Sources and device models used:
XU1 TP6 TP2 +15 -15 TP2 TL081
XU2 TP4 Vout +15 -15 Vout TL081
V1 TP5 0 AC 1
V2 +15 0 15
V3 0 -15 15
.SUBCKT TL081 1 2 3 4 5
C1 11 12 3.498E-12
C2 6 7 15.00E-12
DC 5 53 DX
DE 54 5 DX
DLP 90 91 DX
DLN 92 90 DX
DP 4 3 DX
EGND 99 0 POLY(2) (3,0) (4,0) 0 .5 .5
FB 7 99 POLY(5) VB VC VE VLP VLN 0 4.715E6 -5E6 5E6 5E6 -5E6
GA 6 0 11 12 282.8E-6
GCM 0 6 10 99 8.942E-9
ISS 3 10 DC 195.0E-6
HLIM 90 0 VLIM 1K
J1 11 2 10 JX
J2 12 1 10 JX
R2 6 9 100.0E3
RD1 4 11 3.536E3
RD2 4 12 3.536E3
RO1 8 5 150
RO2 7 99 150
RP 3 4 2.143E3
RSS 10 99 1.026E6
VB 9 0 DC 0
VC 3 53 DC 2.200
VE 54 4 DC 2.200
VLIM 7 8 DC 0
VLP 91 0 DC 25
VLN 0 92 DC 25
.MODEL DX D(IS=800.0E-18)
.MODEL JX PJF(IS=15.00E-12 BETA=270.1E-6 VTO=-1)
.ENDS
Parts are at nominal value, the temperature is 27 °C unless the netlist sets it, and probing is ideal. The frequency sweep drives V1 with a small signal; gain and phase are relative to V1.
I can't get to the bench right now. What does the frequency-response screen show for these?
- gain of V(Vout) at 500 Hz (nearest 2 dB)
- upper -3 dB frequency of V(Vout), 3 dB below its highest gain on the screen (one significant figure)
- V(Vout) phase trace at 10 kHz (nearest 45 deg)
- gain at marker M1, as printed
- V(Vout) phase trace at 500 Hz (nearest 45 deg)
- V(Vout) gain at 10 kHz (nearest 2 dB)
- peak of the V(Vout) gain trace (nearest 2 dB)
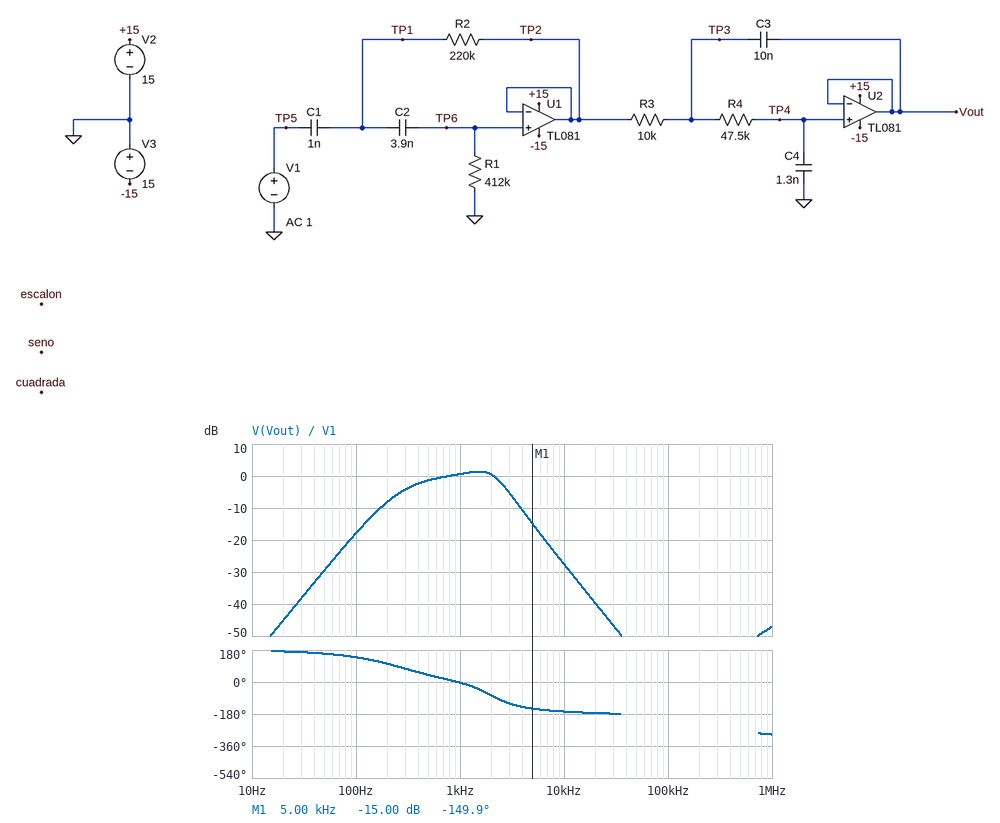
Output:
-2 dB
2 kHz
-180 deg
-15.00 dB
45 deg
-28 dB
2 dB
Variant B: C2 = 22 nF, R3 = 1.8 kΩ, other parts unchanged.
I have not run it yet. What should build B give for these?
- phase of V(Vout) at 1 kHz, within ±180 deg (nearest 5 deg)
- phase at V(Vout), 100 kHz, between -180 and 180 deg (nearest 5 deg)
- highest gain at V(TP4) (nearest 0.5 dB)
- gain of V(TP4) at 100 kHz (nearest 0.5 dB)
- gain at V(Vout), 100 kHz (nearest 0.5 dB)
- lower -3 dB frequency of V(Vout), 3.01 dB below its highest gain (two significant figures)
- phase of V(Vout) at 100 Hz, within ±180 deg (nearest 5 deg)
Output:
0 deg
135 deg
-1.0 dB
-53.0 dB
-49.5 dB
310 Hz
90 deg
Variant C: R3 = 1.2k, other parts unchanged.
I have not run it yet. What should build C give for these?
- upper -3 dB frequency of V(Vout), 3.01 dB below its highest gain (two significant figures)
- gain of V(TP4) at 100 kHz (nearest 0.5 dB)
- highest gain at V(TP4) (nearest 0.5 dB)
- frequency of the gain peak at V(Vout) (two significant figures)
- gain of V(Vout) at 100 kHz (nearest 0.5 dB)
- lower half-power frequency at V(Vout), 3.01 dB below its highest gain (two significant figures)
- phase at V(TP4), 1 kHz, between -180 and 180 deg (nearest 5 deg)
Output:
3.6 kHz
-49.5 dB
-1.0 dB
1.0 kHz
-46.0 dB
320 Hz
5 deg
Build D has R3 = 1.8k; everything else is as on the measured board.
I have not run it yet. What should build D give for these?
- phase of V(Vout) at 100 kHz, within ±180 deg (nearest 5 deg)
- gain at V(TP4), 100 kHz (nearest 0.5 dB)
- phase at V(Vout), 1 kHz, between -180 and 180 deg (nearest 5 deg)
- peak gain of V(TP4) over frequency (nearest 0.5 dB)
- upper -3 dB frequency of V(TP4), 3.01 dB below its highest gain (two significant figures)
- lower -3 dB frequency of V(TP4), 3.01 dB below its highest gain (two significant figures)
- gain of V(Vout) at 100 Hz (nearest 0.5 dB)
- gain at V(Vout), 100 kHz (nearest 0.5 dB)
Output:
135 deg
-53.0 dB
5 deg
-0.5 dB
3.7 kHz
320 Hz
-18.0 dB
-49.5 dB
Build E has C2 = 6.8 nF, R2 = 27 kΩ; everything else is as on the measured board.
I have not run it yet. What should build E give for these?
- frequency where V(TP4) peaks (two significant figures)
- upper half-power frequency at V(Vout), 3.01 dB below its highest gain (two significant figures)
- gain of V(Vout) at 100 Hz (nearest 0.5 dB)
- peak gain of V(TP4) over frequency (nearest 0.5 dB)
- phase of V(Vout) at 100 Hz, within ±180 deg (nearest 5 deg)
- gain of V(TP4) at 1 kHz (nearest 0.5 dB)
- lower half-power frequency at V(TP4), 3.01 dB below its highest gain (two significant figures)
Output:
710 Hz
2.1 kHz
-30.5 dB
3.5 dB
170 deg
3.0 dB
490 Hz
